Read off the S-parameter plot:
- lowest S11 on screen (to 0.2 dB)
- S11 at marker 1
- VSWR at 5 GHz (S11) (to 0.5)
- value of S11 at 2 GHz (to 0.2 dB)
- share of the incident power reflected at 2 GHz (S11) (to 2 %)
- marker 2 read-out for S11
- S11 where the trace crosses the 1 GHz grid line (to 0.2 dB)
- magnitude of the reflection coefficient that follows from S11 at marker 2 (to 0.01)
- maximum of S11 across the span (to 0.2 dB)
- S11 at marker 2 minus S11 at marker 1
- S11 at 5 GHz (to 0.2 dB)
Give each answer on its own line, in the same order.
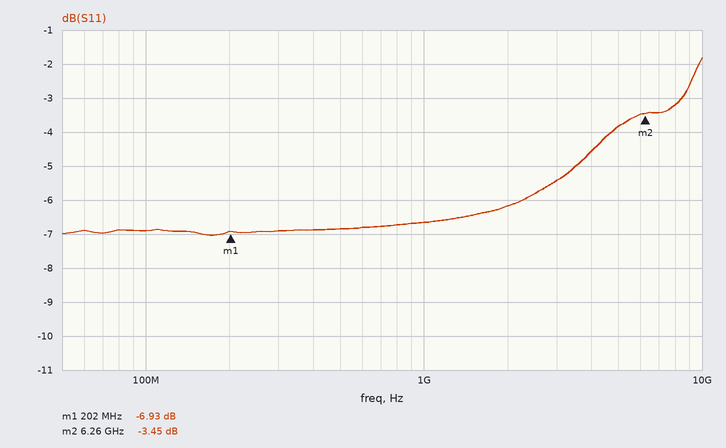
-7.0 dB
-6.93 dB
4.5
-6.2 dB
24 %
-3.45 dB
-6.6 dB
0.67
-1.8 dB
3.48 dB
-3.8 dB
